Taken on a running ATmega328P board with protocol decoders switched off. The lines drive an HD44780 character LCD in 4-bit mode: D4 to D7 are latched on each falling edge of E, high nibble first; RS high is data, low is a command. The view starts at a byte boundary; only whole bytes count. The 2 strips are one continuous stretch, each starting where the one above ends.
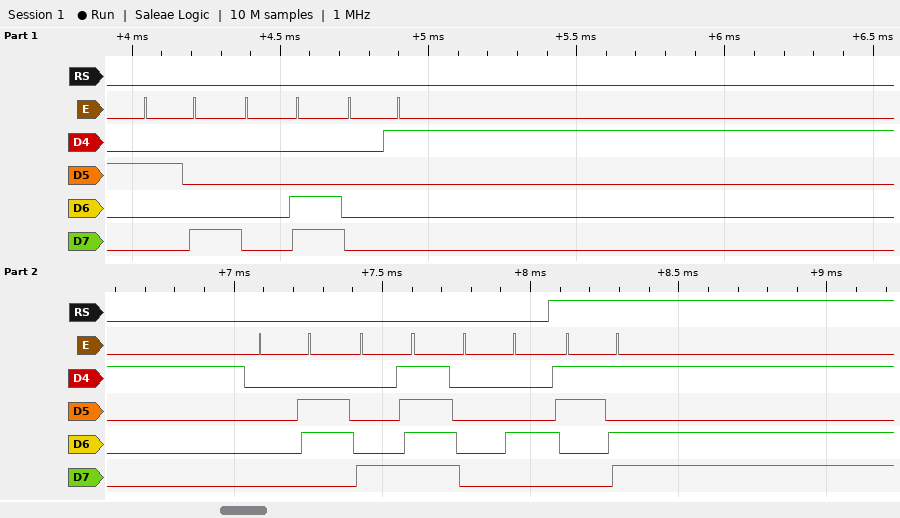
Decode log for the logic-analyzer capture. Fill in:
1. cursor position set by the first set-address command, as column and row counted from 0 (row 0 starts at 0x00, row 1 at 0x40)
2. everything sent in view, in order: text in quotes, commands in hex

column 15, row 0
0x28 0x0C 0x01 0x06 0x8F 0x04 "="
